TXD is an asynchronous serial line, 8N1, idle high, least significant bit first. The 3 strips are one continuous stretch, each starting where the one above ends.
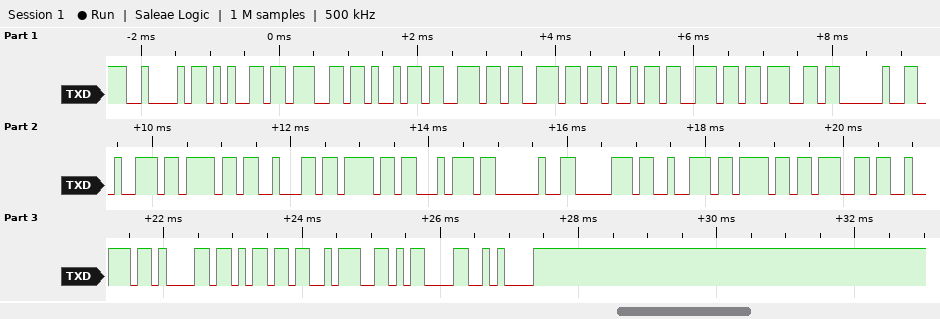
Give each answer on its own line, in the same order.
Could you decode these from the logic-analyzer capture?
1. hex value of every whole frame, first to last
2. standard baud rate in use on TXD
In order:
42 65 67 69 6E 6E 69 6E 67 20 72 6F 62 6F 74 20 70 72 6F 67 72 61 6D 3A 0D 0A
9600 baud
